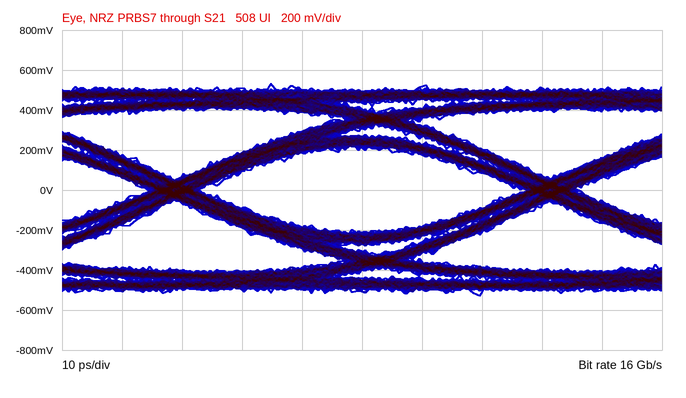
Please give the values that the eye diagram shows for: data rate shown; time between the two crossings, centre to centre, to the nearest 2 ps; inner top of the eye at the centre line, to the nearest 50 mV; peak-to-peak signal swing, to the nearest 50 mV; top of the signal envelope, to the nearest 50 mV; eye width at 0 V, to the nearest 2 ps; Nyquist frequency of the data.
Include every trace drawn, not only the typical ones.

16 Gb/s
62 ps
200 mV
1.05 V
550 mV
54 ps
8 GHz
